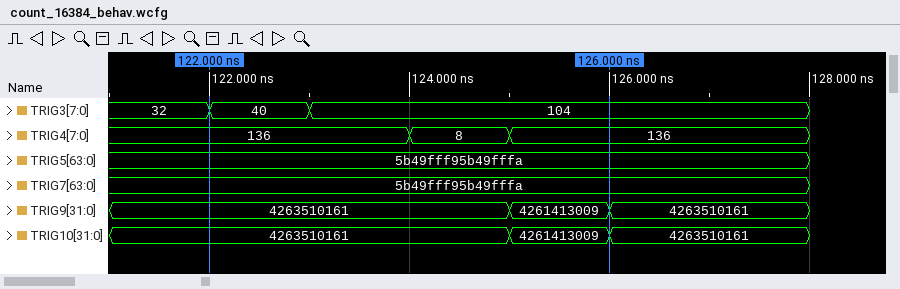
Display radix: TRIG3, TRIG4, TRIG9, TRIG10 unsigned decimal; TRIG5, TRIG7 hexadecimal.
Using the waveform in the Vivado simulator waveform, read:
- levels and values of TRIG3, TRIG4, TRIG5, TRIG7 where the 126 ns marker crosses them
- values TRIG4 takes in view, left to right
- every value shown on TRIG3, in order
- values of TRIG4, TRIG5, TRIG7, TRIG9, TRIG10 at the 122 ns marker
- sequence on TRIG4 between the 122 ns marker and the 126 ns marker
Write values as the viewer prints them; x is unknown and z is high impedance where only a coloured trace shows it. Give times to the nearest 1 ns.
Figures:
TRIG3=104, TRIG4=136, TRIG5=5b49fff95b49fffa, TRIG7=5b49fff95b49fffa
136, 8, 136
32, 40, 104
TRIG4=136, TRIG5=5b49fff95b49fffa, TRIG7=5b49fff95b49fffa, TRIG9=4263510161, TRIG10=4263510161
136, 8, 136
